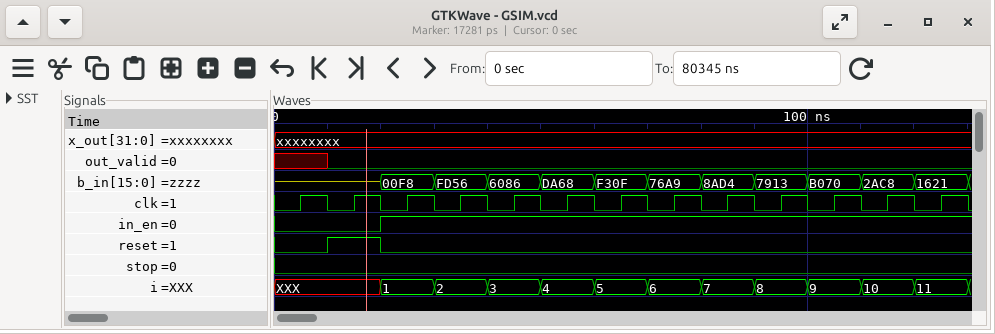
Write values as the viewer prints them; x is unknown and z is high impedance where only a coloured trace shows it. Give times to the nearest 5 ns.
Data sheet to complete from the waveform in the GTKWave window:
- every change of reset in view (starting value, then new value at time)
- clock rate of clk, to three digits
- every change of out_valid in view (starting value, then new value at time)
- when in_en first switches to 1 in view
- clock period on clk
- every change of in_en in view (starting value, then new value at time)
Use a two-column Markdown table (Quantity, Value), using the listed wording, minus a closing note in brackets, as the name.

| Quantity | Value |
|---|---|
| every change of reset in view | 0, 1 at 10 ns, 0 at 20 ns |
| clock rate of clk, to three digits | 100 MHz |
| every change of out_valid in view | x, 0 at 10 ns |
| when in_en first switches to 1 in view | 20 ns |
| clock period on clk | 10 ns |
| every change of in_en in view | 0, 1 at 20 ns |
